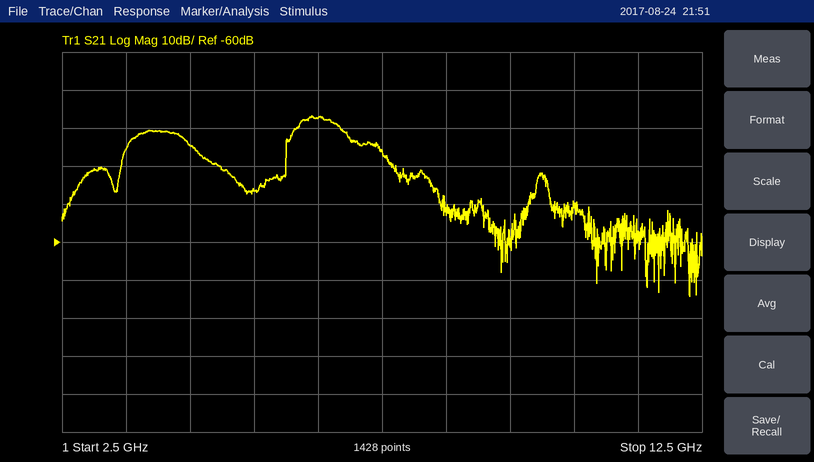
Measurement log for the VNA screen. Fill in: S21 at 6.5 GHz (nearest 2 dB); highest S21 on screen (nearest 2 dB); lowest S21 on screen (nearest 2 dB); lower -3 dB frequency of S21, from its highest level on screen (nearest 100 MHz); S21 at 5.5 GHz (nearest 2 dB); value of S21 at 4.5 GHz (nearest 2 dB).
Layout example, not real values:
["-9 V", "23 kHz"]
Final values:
["-28 dB", "-26 dB", "-74 dB", "6.2 GHz", "-46 dB", "-34 dB"]
